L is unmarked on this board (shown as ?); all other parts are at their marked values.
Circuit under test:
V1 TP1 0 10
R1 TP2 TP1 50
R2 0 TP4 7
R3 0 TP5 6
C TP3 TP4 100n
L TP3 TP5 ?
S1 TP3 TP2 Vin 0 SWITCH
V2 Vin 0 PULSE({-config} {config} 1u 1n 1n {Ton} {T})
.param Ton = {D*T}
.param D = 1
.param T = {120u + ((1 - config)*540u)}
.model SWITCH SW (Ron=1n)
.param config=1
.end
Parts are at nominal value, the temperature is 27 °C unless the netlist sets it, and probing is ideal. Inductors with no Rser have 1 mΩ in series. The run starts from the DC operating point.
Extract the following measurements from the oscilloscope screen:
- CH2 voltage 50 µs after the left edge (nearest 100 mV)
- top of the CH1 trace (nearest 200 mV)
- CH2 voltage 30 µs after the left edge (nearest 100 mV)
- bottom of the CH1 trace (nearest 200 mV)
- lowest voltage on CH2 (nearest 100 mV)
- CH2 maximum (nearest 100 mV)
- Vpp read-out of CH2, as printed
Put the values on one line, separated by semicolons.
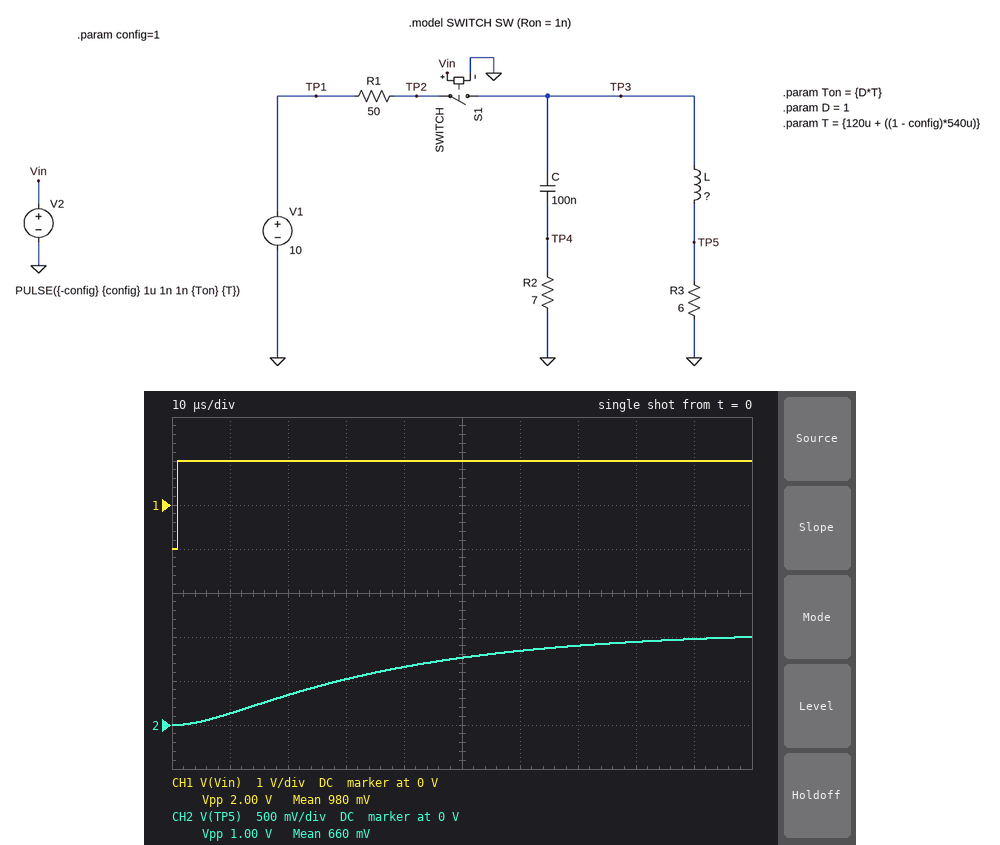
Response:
800 mV; 1.0 V; 500 mV; -1.0 V; 0 V; 1.0 V; 1.00 V
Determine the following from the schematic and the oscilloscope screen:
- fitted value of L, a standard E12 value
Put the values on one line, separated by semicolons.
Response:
2.2 mH
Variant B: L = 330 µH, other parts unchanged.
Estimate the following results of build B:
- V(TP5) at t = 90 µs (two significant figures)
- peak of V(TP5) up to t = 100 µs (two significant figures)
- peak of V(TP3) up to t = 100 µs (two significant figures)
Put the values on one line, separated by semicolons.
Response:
1.1 V; 1.2 V; 5.5 V
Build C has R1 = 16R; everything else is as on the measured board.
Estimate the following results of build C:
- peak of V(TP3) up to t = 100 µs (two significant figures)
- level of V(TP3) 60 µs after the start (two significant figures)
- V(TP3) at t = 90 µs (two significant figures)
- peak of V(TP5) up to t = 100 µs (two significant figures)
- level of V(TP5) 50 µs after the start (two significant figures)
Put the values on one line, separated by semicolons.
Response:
9.4 V; 6.9 V; 5.8 V; 1.7 V; 1.0 V
